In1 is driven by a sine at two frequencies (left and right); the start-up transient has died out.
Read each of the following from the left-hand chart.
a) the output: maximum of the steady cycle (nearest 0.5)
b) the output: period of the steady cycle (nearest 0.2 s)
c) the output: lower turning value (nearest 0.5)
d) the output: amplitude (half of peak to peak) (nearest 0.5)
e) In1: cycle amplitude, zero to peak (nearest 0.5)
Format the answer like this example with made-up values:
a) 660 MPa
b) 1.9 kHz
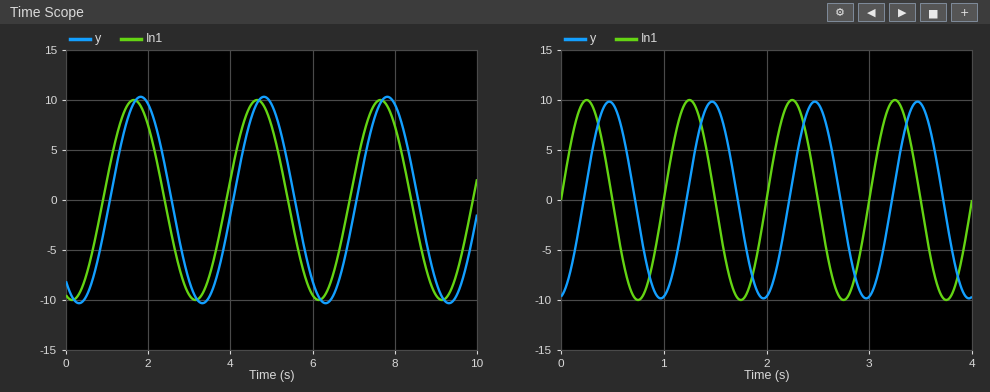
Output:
a) 10.5
b) 3.0 s
c) -10.5
d) 10.5
e) 10.0
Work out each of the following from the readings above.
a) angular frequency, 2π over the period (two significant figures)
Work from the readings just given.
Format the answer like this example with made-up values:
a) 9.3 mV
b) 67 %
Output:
a) 2.1 rad/s
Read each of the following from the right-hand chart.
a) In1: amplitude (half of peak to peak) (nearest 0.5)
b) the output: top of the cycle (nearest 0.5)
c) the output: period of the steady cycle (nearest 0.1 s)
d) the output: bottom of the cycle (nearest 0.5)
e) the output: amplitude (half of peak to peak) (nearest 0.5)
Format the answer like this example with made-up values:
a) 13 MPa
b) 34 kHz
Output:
a) 10.0
b) 10.0
c) 1.0 s
d) -10.0
e) 10.0
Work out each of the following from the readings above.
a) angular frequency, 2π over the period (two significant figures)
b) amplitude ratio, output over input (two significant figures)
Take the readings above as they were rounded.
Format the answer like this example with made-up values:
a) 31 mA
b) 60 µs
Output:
a) 6.3 rad/s
b) 1.0
